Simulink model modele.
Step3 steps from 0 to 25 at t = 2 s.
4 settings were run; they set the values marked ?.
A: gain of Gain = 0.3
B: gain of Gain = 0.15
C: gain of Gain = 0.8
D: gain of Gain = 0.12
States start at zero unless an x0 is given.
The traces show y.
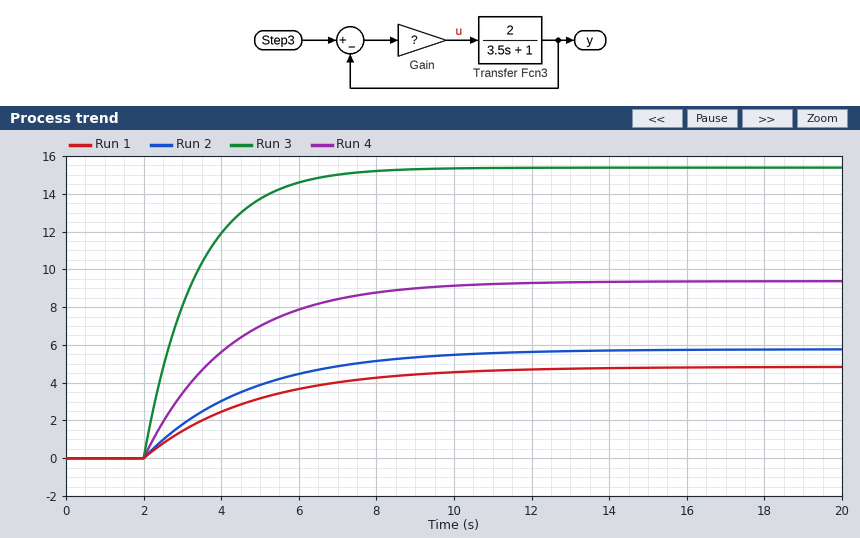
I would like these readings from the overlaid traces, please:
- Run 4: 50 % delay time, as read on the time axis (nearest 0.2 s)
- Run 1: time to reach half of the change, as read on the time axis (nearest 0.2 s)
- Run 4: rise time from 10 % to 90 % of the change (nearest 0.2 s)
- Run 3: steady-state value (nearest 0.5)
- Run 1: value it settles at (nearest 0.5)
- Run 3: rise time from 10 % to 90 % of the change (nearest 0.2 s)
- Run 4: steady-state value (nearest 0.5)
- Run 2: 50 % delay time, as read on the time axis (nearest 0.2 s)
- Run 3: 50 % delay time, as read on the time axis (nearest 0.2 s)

3.6 s
4.0 s
4.8 s
15.5
5.0
3.0 s
9.5
3.8 s
3.0 s
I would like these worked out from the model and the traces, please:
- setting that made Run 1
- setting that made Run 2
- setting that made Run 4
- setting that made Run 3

D
B
A
C
